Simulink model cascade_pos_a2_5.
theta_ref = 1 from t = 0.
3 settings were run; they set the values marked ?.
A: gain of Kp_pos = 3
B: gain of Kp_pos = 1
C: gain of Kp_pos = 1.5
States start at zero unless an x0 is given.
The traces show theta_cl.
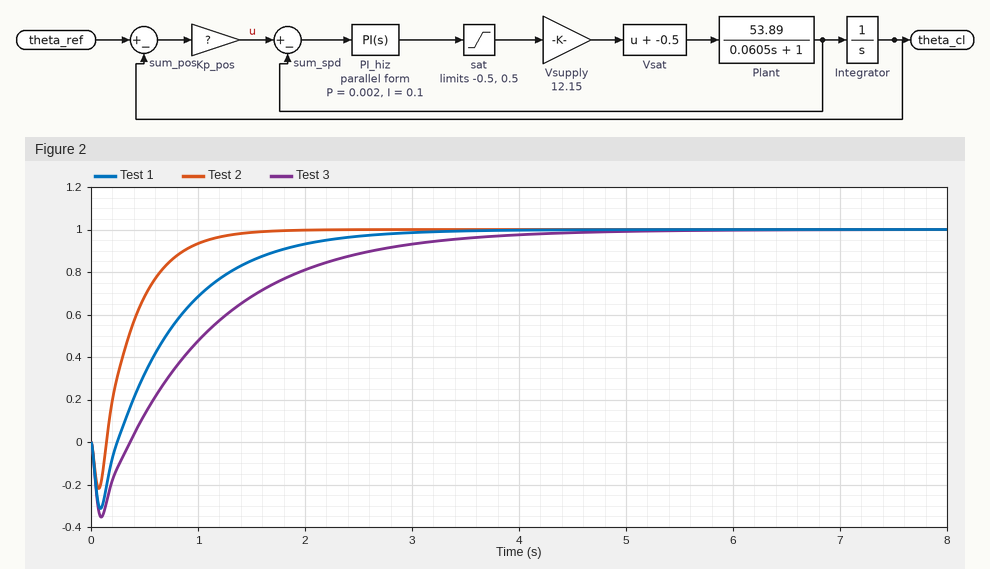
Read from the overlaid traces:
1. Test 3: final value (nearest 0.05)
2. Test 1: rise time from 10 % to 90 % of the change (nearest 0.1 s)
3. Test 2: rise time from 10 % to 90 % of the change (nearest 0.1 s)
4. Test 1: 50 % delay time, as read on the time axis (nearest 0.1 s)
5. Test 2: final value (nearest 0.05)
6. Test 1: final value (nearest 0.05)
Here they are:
1.00
1.4 s
0.7 s
0.7 s
1.00
1.00
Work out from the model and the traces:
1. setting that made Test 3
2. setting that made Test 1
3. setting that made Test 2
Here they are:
B
C
A
